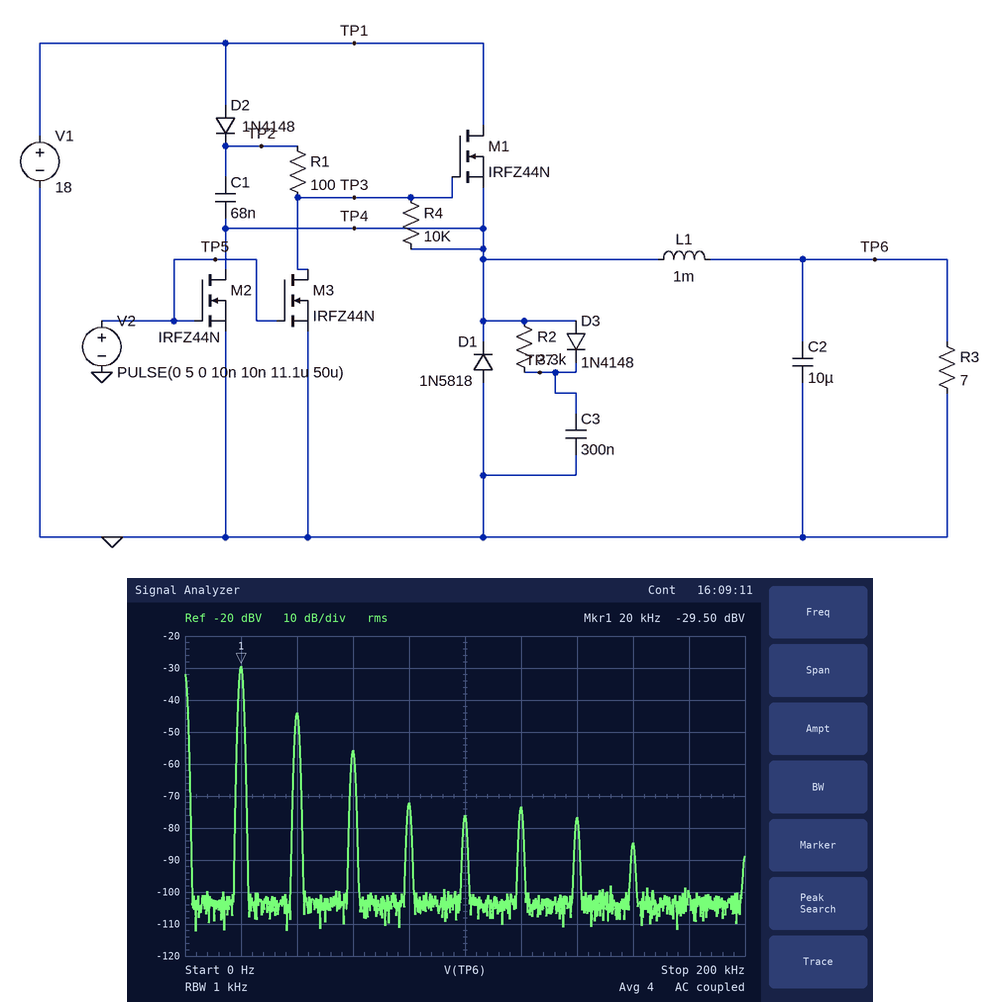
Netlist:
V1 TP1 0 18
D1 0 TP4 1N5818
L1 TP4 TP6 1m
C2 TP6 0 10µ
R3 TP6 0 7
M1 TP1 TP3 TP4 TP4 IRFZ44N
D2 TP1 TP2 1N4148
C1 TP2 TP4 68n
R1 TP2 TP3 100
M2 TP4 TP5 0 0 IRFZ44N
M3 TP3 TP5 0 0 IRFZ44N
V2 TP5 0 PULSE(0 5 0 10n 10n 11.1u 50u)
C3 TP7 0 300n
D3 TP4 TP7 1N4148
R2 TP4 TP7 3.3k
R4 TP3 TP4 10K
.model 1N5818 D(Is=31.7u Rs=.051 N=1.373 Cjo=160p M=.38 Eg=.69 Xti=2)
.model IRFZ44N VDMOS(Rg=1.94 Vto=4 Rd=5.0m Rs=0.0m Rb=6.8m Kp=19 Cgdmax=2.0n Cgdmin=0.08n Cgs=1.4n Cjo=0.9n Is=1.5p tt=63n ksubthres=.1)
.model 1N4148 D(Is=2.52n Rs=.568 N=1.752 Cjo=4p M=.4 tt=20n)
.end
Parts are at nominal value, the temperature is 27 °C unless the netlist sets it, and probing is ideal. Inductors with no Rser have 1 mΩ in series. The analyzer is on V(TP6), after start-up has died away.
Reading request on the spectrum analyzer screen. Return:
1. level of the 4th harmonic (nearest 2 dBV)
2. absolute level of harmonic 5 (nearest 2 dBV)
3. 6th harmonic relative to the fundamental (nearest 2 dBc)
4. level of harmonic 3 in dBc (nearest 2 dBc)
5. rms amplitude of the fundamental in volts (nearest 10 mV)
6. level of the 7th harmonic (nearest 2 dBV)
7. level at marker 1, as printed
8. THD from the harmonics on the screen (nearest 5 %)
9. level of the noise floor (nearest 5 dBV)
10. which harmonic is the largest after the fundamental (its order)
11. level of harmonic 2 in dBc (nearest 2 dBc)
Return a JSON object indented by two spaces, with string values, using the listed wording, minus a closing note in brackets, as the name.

{
  "level of the 4th harmonic": "-72 dBV",
  "absolute level of harmonic 5": "-76 dBV",
  "6th harmonic relative to the fundamental": "-44 dBc",
  "level of harmonic 3 in dBc": "-26 dBc",
  "rms amplitude of the fundamental in volts": "30 mV",
  "level of the 7th harmonic": "-76 dBV",
  "level at marker 1, as printed": "-29.50 dBV",
  "THD from the harmonics on the screen": "20 %",
  "level of the noise floor": "-105 dBV",
  "which harmonic is the largest after the fundamental": "2",
  "level of harmonic 2 in dBc": "-14 dBc"
}
